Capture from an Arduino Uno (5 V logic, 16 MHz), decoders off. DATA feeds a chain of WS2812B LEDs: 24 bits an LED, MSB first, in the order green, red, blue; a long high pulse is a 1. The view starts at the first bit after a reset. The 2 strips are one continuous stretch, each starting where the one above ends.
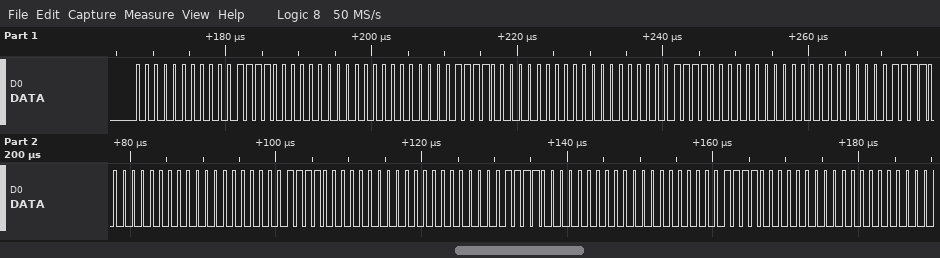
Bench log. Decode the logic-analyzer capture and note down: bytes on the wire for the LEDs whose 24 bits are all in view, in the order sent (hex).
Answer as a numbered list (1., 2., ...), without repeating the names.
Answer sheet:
1. 00 1E 00 00 1E 00 00 1E 00 00 1E 00 00 1E 00 00 1E 00 00 1E 00
